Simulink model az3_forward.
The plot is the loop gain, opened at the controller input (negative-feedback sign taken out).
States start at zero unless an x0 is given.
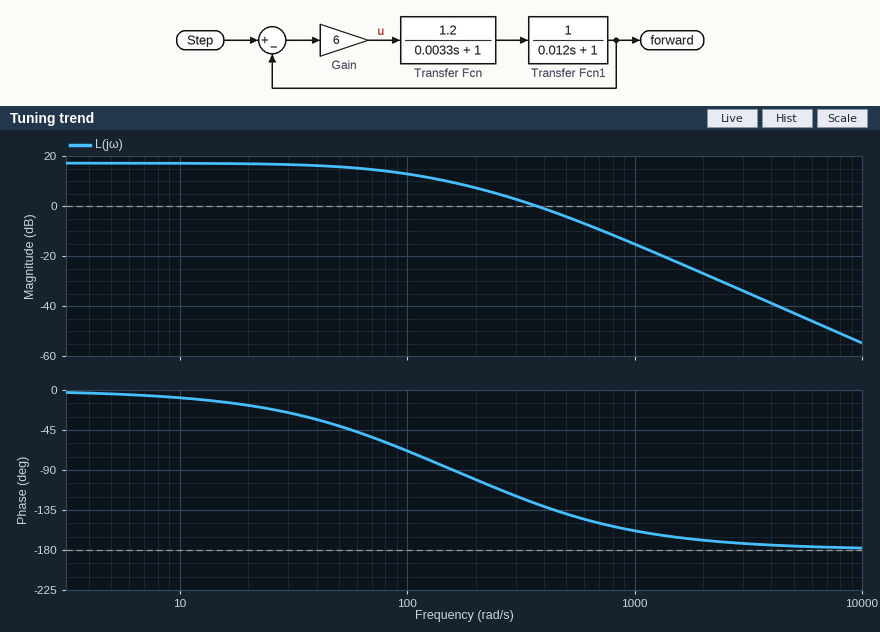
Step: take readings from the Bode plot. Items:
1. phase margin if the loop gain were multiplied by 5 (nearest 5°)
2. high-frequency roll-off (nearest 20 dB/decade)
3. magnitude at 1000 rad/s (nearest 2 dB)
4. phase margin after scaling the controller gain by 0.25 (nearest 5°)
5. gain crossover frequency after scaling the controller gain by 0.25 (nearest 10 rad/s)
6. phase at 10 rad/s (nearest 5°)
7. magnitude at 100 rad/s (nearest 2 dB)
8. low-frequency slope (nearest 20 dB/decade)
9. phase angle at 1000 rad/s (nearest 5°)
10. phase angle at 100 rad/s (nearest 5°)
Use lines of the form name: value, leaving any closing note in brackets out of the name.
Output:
phase margin if the loop gain were multiplied by 5: 25°
high-frequency roll-off: -40 dB/decade
magnitude at 1000 rad/s: -16 dB
phase margin after scaling the controller gain by 0.25: 105°
gain crossover frequency after scaling the controller gain by 0.25: 110 rad/s
phase at 10 rad/s: -10°
magnitude at 100 rad/s: 12 dB
low-frequency slope: 0 dB/decade
phase angle at 1000 rad/s: -160°
phase angle at 100 rad/s: -70°
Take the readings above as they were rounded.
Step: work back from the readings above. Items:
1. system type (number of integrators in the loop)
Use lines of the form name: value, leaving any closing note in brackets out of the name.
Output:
system type: 0
